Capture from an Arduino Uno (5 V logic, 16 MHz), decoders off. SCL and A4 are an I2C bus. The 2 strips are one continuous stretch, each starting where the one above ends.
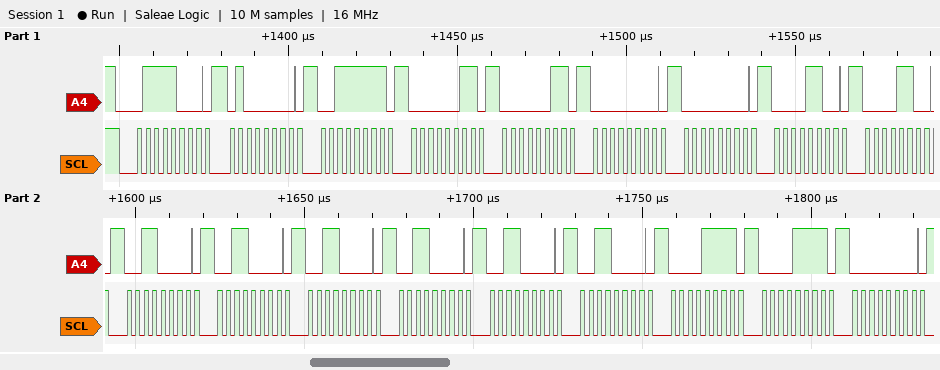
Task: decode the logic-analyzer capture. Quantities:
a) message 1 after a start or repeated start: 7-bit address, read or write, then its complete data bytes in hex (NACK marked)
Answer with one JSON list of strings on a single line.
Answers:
["0x3C write: 40 3F 03 03 00 00 0C 0C 30 30 30 30 30 30 0F 0F 00"]
